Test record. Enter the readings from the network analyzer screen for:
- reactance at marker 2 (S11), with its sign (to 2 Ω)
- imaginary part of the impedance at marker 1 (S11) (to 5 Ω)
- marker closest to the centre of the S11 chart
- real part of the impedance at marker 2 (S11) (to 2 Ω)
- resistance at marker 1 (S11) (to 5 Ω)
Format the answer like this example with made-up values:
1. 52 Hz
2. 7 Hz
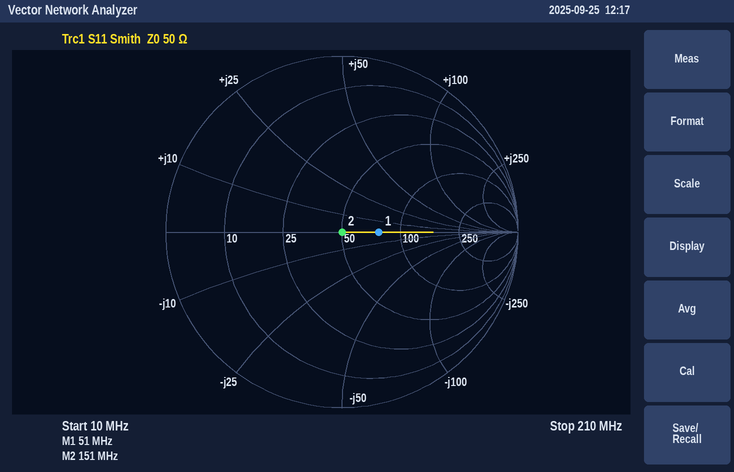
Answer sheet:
1. 0 Ω
2. 0 Ω
3. marker 2
4. 50 Ω
5. 75 Ω
